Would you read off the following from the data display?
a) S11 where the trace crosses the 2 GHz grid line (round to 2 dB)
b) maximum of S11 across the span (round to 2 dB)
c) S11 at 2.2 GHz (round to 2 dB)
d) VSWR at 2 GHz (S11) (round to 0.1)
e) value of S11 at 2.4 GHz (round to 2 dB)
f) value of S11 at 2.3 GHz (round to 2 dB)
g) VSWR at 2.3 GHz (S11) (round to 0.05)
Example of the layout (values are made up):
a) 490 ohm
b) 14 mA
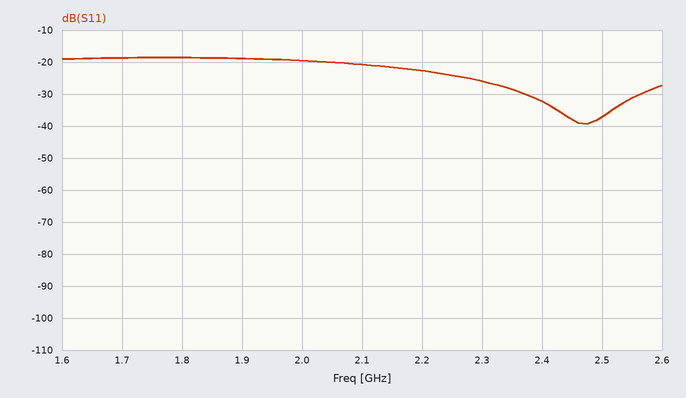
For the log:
a) -20 dB
b) -18 dB
c) -22 dB
d) 1.2
e) -32 dB
f) -26 dB
g) 1.10
